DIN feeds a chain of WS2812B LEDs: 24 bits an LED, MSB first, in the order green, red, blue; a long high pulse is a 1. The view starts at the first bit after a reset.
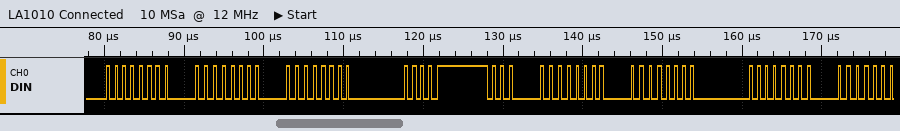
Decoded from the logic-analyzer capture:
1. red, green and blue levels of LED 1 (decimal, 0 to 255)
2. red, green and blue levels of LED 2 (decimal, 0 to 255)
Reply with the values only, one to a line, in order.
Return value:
0, 0, 0
0, 8, 0
